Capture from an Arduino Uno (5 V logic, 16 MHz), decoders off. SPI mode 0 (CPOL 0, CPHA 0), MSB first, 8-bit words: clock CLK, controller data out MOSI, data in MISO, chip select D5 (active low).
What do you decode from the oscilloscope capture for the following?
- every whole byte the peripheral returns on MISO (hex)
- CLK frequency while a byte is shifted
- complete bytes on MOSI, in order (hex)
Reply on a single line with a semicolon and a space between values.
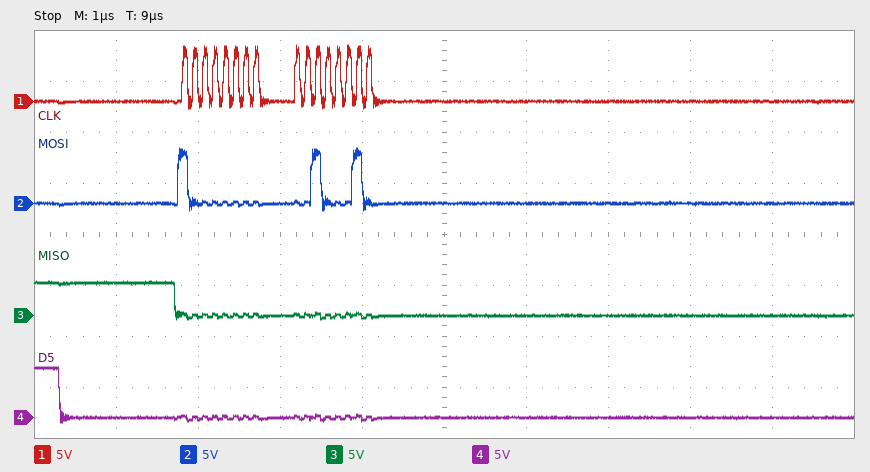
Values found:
00 00; 8 MHz; 80 22
